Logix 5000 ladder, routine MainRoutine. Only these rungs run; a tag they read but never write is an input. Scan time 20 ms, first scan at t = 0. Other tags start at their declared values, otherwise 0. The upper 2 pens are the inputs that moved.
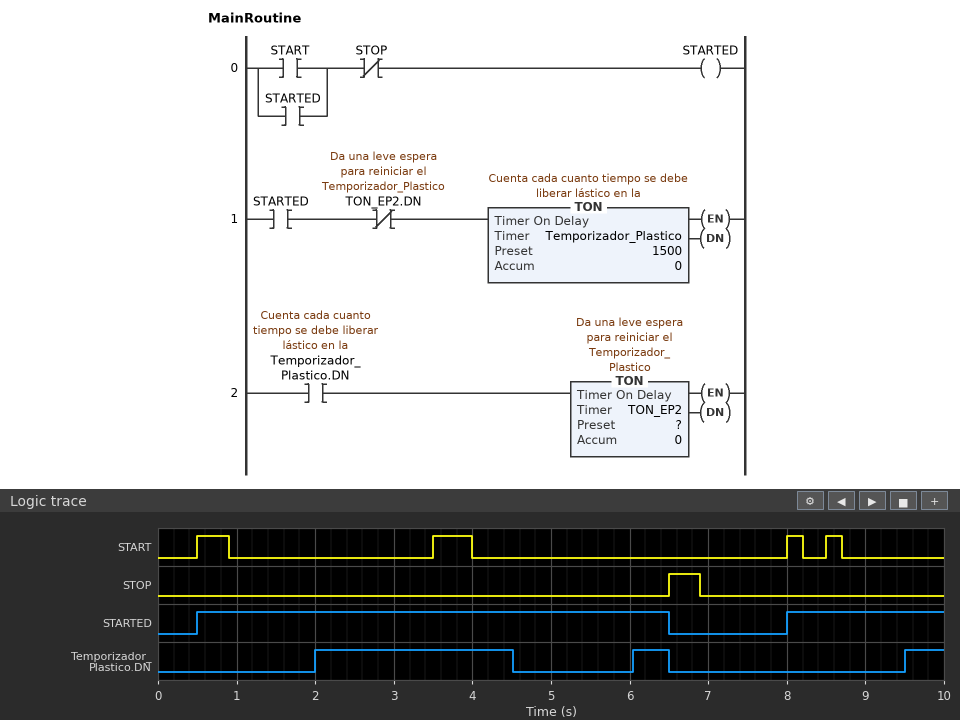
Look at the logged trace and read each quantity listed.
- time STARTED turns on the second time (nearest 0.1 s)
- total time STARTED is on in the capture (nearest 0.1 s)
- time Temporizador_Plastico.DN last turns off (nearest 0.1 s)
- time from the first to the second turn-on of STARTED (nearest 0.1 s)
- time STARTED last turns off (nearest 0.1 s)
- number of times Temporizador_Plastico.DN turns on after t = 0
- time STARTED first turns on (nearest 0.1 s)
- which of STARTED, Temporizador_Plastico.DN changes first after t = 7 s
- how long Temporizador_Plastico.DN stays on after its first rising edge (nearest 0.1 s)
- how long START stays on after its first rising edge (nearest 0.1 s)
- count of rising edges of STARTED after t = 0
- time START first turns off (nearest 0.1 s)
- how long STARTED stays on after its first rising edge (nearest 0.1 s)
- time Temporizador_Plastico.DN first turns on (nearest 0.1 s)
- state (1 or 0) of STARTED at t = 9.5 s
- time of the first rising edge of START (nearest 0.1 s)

8.0 s
8.0 s
6.5 s
7.5 s
6.5 s
3
0.5 s
STARTED
2.5 s
0.4 s
2
0.9 s
6.0 s
2.0 s
1
0.5 s
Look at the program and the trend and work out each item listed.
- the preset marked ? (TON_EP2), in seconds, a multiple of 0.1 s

2.5 s
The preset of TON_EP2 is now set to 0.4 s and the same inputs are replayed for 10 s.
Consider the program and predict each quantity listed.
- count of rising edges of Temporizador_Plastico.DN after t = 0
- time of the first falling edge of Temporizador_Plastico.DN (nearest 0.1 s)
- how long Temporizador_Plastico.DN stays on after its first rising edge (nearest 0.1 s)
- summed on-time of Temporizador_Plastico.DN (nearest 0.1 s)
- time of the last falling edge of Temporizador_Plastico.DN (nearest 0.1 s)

4
2.4 s
0.4 s
1.7 s
9.9 s
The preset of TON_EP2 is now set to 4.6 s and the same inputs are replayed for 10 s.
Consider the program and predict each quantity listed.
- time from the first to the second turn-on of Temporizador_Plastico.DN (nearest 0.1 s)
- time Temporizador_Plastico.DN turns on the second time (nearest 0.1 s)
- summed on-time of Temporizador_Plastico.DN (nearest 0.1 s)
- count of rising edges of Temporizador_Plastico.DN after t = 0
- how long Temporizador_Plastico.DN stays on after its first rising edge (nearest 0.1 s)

7.5 s
9.5 s
5.0 s
2
4.5 s
